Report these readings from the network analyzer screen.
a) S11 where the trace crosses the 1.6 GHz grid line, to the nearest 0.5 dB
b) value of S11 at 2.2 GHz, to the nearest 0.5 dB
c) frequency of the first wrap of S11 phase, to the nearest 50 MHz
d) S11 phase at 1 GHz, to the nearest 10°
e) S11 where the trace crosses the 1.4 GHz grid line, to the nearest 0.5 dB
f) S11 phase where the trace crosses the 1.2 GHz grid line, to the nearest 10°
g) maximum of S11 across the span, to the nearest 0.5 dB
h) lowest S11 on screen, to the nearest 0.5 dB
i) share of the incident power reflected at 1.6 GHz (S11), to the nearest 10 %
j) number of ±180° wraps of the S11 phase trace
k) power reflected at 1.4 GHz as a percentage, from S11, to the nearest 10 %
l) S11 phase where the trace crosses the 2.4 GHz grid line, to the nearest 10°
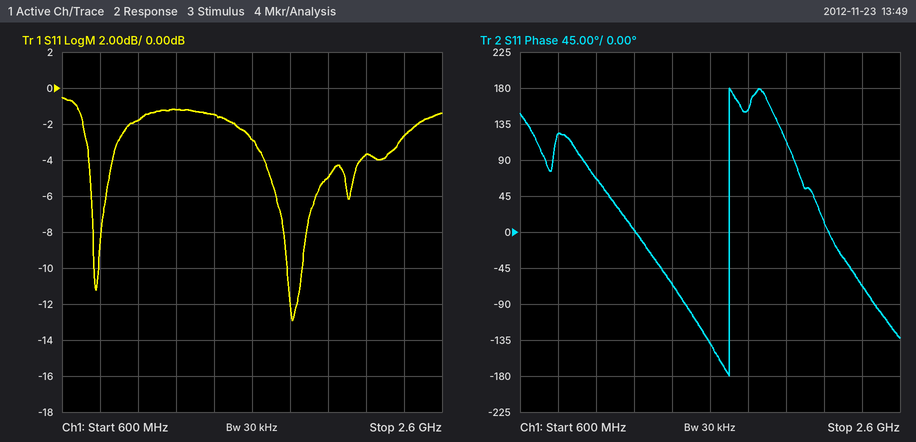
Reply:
-3.0 dB
-3.5 dB
1.70 GHz
70°
-1.5 dB
0°
-0.5 dB
-13.0 dB
50 %
1
70 %
-70°
